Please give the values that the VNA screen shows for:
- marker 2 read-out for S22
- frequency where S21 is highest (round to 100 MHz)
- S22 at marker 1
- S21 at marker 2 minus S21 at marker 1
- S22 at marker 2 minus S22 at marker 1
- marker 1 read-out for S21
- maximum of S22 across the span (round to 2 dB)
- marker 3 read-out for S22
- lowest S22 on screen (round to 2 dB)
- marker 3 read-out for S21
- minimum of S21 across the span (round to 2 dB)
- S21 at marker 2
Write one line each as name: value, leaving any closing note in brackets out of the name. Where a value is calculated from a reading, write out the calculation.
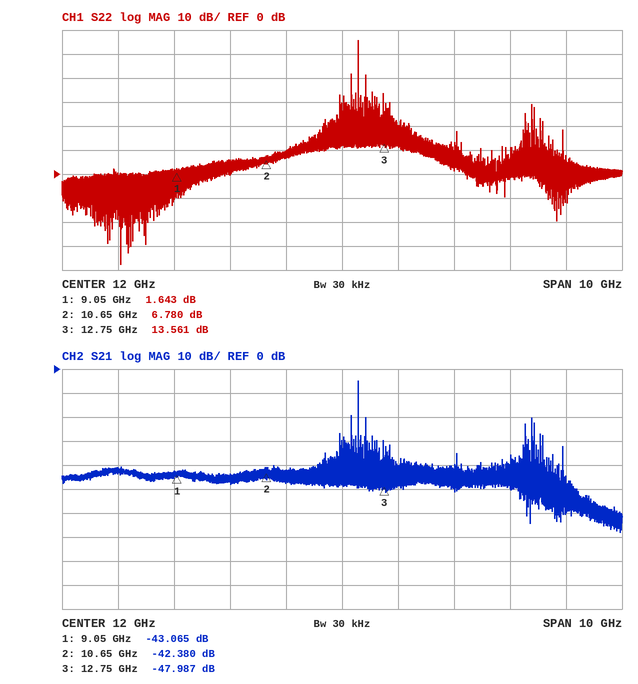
marker 2 read-out for S22: 6.780 dB
frequency where S21 is highest: 12.3 GHz
S22 at marker 1: 1.643 dB
S21 at marker 2 minus S21 at marker 1: -42.38 − (-43.065) = 0.685 dB
S22 at marker 2 minus S22 at marker 1: 6.78 − (1.643) = 5.137 dB
marker 1 read-out for S21: -43.065 dB
maximum of S22 across the span: 56 dB
marker 3 read-out for S22: 13.561 dB
lowest S22 on screen: -38 dB
marker 3 read-out for S21: -47.987 dB
minimum of S21 across the span: -68 dB
S21 at marker 2: -42.380 dB
